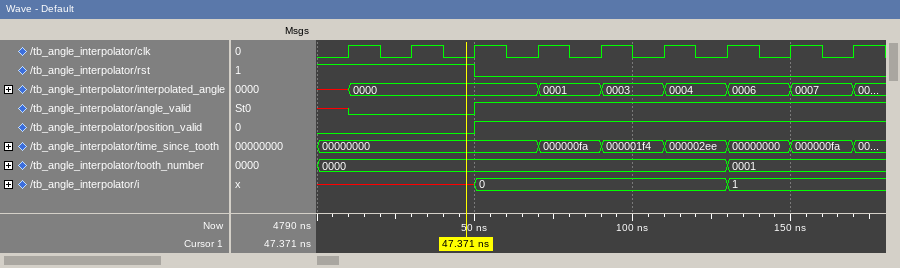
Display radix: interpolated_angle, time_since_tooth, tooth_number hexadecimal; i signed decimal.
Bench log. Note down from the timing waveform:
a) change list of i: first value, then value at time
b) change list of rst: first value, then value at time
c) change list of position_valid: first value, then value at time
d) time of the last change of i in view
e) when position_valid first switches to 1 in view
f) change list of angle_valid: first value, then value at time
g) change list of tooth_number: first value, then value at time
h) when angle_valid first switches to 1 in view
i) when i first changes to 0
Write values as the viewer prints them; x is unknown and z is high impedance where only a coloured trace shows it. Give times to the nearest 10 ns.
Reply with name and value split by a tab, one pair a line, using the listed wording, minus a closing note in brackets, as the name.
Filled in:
change list of i: first value, then value at time	x, 0 at 50 ns, 1 at 130 ns
change list of rst: first value, then value at time	1, 0 at 50 ns
change list of position_valid: first value, then value at time	0, 1 at 50 ns
time of the last change of i in view	130 ns
when position_valid first switches to 1 in view	50 ns
change list of angle_valid: first value, then value at time	x, 0 at 10 ns, 1 at 50 ns
change list of tooth_number: first value, then value at time	0000, 0001 at 130 ns
when angle_valid first switches to 1 in view	50 ns
when i first changes to 0	50 ns
